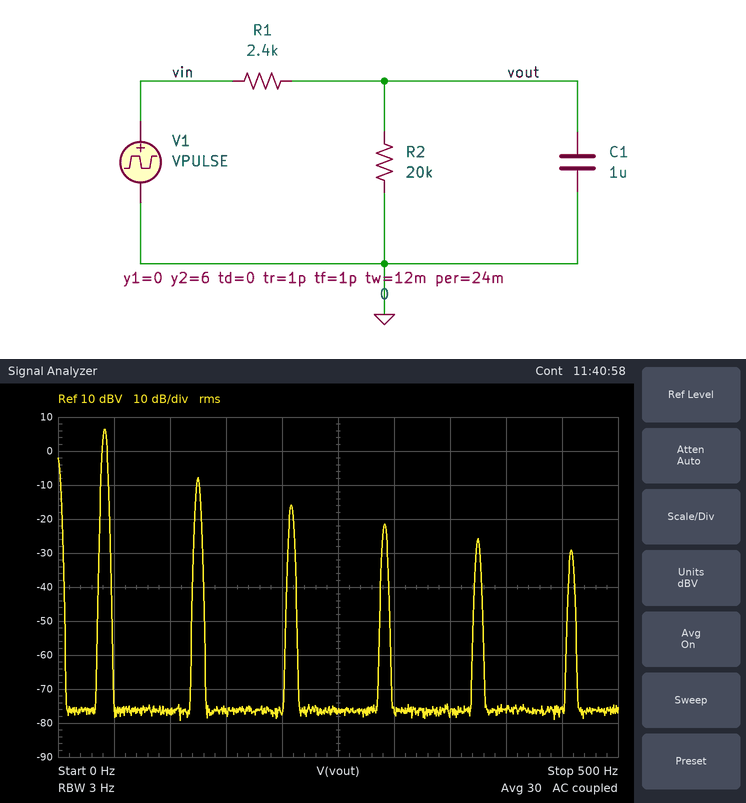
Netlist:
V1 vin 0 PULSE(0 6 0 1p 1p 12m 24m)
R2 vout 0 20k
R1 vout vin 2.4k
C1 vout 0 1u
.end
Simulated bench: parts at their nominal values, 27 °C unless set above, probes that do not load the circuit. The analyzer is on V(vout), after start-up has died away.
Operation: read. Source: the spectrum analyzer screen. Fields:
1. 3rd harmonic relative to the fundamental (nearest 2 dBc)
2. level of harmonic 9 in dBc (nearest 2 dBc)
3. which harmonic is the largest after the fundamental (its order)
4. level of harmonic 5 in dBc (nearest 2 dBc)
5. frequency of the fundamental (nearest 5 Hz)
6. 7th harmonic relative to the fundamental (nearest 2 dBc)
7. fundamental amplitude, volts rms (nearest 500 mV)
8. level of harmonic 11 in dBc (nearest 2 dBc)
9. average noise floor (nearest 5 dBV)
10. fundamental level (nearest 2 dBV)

-14 dBc
-32 dBc
3
-22 dBc
40 Hz
-28 dBc
2.0 V
-36 dBc
-75 dBV
6 dBV
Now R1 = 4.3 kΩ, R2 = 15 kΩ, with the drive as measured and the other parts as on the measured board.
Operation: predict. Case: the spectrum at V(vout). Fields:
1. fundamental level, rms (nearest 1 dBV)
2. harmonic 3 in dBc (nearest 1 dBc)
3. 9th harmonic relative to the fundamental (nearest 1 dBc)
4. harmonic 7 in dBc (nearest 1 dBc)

4 dBV
-16 dBc
-35 dBc
-30 dBc
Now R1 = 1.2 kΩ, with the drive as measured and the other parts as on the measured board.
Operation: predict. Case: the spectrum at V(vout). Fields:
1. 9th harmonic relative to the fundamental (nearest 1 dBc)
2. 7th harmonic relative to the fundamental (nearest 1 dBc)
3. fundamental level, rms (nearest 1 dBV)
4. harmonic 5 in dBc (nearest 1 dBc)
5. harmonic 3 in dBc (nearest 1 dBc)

-28 dBc
-24 dBc
8 dBV
-19 dBc
-12 dBc
